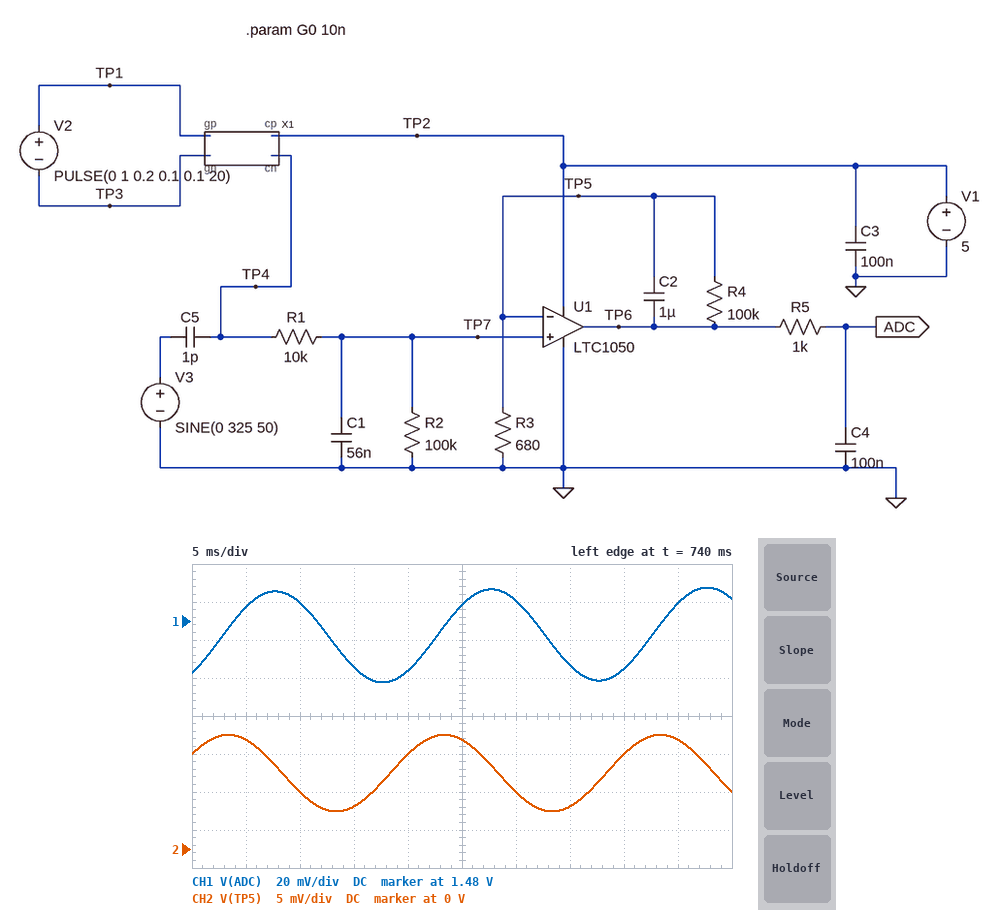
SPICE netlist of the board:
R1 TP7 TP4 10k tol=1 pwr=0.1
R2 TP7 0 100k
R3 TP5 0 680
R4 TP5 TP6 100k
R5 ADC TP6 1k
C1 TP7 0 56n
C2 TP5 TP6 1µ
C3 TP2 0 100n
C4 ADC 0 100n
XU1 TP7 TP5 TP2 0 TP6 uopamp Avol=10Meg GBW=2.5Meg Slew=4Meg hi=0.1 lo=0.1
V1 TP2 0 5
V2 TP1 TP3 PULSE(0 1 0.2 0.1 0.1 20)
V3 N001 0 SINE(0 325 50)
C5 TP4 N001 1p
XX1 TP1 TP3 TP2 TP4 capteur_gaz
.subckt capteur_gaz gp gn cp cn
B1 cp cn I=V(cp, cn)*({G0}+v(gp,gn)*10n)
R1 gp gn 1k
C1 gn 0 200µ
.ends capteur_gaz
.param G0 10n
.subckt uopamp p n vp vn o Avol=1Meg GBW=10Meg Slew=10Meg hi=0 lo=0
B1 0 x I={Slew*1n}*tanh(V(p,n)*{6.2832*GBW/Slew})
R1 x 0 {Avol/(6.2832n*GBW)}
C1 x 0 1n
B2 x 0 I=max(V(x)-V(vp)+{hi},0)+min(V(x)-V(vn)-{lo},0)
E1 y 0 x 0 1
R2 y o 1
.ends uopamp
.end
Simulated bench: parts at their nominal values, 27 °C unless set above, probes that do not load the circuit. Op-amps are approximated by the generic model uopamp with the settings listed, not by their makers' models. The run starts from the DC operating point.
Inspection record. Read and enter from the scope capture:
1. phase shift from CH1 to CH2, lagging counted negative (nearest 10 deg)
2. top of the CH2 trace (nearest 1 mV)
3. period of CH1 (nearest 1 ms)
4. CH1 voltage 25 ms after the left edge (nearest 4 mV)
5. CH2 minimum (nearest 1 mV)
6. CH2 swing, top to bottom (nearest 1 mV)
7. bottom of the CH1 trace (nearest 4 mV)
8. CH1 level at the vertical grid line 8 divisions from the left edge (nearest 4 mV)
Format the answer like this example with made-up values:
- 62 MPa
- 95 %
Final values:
- 80 deg
- 15 mV
- 20 ms
- 1.488 V
- 5 mV
- 10 mV
- 1.448 V
- 1.456 V
